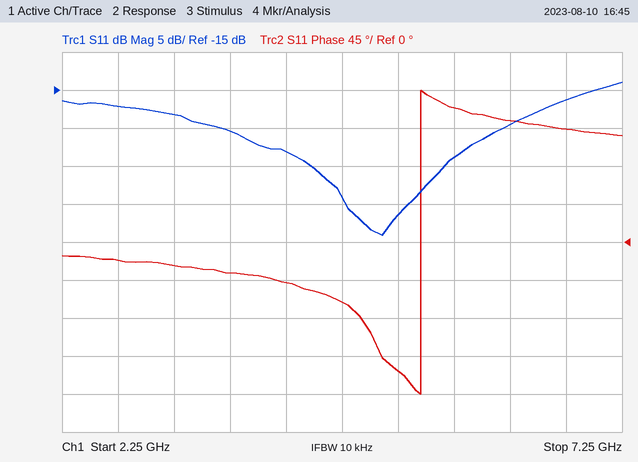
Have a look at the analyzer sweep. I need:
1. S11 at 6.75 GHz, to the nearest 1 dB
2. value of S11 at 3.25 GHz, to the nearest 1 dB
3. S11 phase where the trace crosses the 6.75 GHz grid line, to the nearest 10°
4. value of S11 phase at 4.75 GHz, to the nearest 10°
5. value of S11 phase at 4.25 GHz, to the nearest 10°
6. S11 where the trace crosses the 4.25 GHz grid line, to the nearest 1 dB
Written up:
-16 dB
-18 dB
130°
-70°
-50°
-23 dB
